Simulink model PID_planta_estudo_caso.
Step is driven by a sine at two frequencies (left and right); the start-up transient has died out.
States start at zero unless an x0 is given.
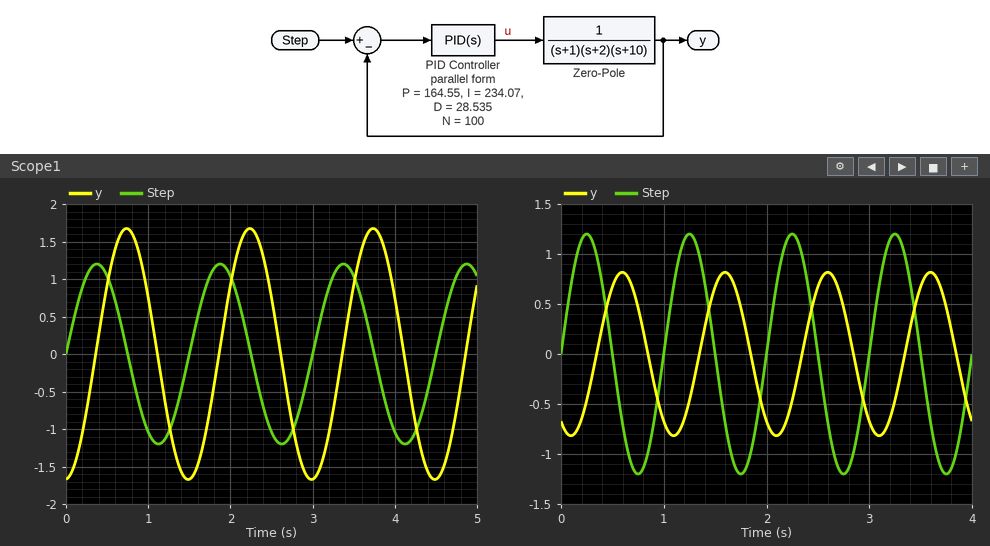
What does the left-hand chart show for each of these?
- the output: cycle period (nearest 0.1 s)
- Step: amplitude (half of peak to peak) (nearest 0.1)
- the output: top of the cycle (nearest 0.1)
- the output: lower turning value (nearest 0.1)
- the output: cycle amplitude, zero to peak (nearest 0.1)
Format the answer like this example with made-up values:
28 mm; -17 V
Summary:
1.5 s; 1.2; 1.7; -1.7; 1.7
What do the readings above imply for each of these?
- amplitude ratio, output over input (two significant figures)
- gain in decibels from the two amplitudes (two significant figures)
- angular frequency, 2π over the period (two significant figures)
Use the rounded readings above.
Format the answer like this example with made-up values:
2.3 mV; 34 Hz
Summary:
1.4; 3.0 dB; 4.2 rad/s
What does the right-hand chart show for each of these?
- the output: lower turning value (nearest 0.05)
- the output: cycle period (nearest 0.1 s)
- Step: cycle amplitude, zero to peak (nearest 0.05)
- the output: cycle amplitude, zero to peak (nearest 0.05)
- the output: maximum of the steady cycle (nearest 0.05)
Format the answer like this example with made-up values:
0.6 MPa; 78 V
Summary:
-0.80; 1.0 s; 1.20; 0.80; 0.80
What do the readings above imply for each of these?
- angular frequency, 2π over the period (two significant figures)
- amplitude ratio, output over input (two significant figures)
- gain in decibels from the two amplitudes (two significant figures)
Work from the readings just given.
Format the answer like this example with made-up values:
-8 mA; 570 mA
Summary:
6.3 rad/s; 0.67; -3.5 dB
